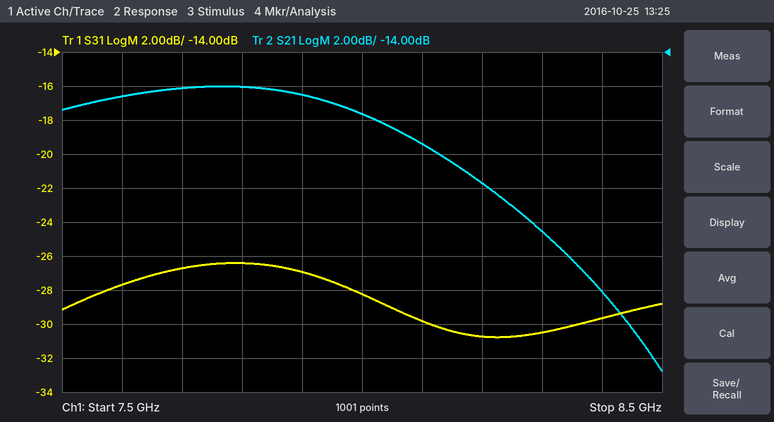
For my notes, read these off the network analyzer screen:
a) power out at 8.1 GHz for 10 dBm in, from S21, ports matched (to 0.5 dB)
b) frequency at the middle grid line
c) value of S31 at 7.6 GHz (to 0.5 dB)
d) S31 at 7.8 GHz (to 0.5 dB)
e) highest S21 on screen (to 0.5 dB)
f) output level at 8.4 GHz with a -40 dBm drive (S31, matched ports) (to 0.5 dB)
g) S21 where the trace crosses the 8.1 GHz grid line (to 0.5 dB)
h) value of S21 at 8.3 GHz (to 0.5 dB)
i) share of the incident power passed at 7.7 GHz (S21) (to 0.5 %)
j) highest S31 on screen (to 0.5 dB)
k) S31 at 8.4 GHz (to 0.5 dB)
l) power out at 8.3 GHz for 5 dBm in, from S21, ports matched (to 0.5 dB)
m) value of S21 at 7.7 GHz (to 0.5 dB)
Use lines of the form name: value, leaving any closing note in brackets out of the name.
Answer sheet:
power out at 8.1 GHz for 10 dBm in, from S21, ports matched: -9.5 dBm
frequency at the middle grid line: 8 GHz
value of S31 at 7.6 GHz: -27.5 dB
S31 at 7.8 GHz: -26.5 dB
highest S21 on screen: -16.0 dB
output level at 8.4 GHz with a -40 dBm drive (S31, matched ports): -69.5 dBm
S21 where the trace crosses the 8.1 GHz grid line: -19.5 dB
value of S21 at 8.3 GHz: -24.5 dB
share of the incident power passed at 7.7 GHz (S21): 2.5 %
highest S31 on screen: -26.5 dB
S31 at 8.4 GHz: -29.5 dB
power out at 8.3 GHz for 5 dBm in, from S21, ports matched: -19.5 dBm
value of S21 at 7.7 GHz: -16.0 dB
